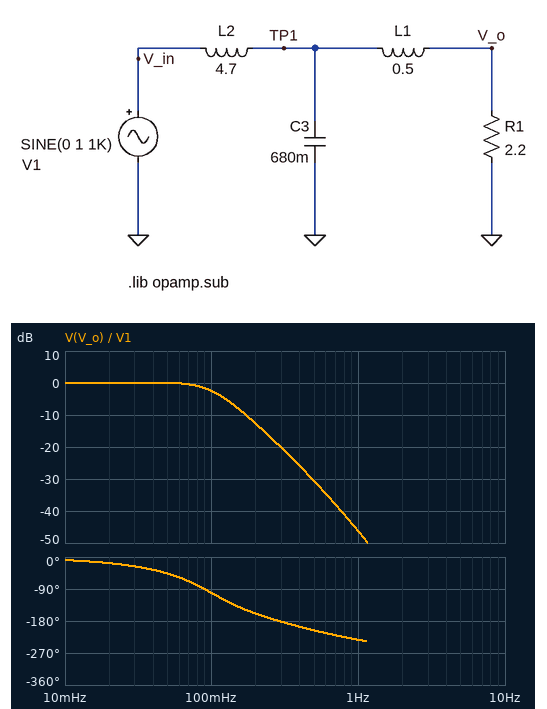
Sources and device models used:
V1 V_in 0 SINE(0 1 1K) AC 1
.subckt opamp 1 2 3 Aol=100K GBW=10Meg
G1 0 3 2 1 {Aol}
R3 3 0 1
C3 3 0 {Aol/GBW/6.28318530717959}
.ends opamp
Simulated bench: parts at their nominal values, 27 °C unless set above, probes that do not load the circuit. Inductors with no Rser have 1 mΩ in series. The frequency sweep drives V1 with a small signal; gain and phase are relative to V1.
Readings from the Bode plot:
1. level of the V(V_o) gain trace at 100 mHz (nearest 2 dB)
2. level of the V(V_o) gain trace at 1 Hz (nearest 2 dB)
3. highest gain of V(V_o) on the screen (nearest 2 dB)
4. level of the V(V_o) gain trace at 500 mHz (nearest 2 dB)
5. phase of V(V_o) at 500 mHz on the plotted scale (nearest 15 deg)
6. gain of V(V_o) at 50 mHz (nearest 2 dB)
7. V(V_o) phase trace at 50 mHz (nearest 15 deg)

-2 dB
-46 dB
0 dB
-30 dB
-210 deg
0 dB
-45 deg
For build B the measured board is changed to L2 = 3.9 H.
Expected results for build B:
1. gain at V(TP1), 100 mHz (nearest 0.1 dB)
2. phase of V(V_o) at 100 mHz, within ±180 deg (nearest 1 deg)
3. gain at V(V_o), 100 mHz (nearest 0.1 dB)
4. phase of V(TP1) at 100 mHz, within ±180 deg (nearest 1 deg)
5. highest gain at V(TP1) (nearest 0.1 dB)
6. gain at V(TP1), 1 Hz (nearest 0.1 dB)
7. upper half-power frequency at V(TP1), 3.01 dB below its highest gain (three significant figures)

-0.8 dB
-92 deg
-0.9 dB
-84 deg
0.4 dB
-39.9 dB
121 mHz
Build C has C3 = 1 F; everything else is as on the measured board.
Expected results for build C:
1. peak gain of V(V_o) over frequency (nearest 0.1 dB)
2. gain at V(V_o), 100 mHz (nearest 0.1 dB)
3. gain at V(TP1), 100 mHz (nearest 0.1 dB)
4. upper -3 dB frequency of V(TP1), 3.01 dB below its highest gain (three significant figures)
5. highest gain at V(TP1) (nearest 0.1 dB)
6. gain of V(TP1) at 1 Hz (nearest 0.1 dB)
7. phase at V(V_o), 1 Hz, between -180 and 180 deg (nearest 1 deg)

1.0 dB
-3.5 dB
-3.4 dB
90.6 mHz
1.1 dB
-45.0 dB
126 deg
